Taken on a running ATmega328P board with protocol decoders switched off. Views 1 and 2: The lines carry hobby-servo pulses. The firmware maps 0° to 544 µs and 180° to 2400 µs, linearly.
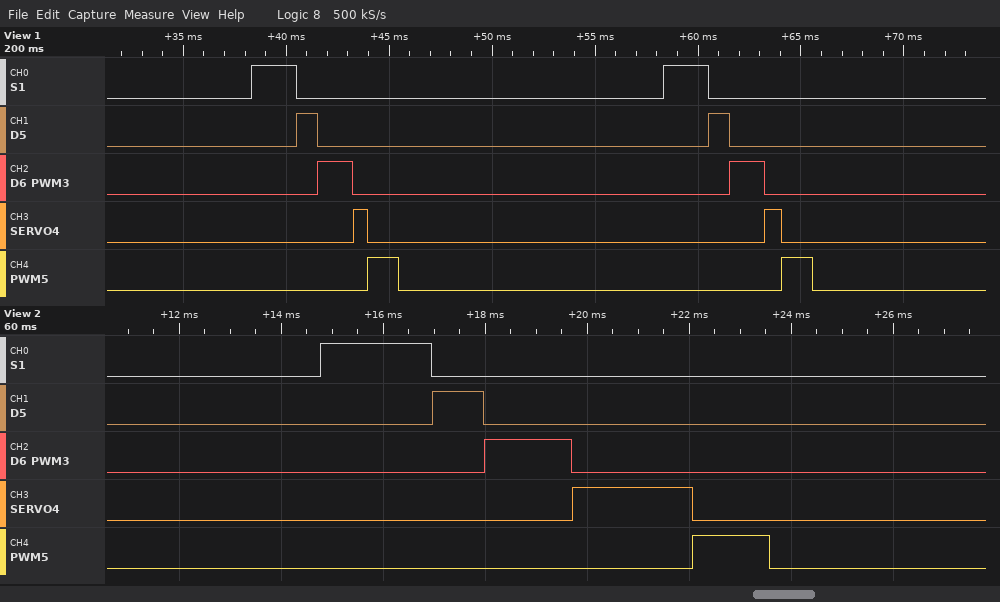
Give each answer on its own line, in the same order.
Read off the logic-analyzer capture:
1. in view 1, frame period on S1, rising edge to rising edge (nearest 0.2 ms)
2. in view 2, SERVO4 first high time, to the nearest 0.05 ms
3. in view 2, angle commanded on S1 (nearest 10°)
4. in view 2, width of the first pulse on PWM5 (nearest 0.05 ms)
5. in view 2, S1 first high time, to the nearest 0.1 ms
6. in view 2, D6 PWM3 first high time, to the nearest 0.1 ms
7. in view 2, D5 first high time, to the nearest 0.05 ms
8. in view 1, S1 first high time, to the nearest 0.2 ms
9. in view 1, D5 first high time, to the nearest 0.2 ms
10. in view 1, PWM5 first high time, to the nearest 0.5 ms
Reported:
20.0 ms
2.35 ms
160°
1.50 ms
2.2 ms
1.7 ms
1.00 ms
2.2 ms
1.0 ms
1.5 ms
